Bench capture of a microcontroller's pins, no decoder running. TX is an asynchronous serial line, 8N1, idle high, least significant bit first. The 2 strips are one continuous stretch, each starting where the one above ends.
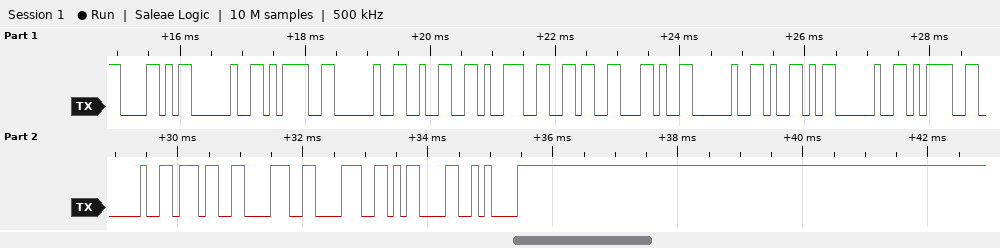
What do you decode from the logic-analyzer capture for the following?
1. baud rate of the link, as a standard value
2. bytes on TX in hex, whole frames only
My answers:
9600 baud
58 20 3D 20 32 39 36 2C 20 59 20 3D 20 37 38 38 0D 0A
